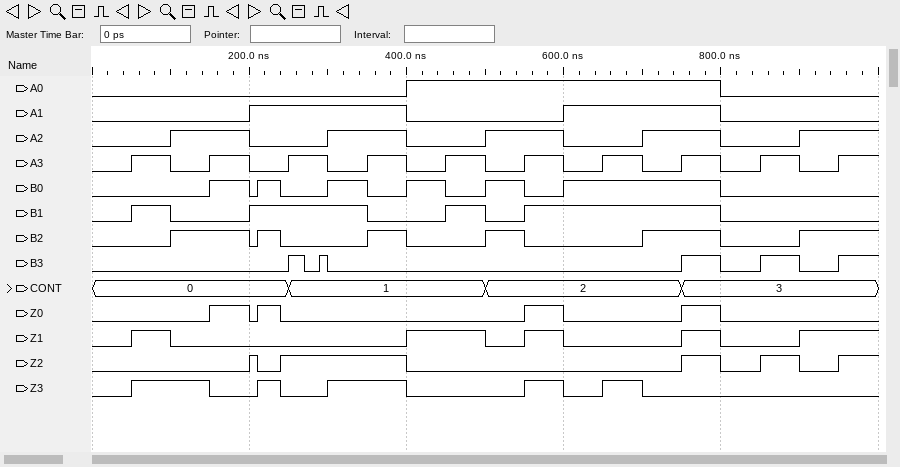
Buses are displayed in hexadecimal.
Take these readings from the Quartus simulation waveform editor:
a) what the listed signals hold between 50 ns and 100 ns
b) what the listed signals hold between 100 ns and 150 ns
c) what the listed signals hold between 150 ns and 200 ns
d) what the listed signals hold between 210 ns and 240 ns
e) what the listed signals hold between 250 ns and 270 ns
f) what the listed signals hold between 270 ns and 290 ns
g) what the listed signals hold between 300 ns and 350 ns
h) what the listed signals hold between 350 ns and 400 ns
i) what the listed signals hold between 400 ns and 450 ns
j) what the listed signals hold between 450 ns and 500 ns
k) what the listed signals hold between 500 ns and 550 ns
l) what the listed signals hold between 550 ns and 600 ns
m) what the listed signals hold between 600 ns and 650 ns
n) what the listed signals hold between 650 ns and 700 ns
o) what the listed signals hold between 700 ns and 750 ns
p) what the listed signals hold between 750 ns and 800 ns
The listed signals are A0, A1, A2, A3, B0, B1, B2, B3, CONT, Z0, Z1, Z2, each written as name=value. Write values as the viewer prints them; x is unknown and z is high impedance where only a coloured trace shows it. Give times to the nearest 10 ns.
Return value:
A0=0, A1=0, A2=0, A3=1, B0=0, B1=1, B2=0, B3=0, CONT=0, Z0=0, Z1=1, Z2=0
A0=0, A1=0, A2=1, A3=0, B0=0, B1=0, B2=1, B3=0, CONT=0, Z0=0, Z1=0, Z2=0
A0=0, A1=0, A2=1, A3=1, B0=1, B1=0, B2=1, B3=0, CONT=0, Z0=1, Z1=0, Z2=0
A0=0, A1=1, A2=0, A3=0, B0=1, B1=1, B2=1, B3=0, CONT=0, Z0=1, Z1=0, Z2=0
A0=0, A1=1, A2=0, A3=1, B0=0, B1=1, B2=0, B3=1, CONT=1, Z0=0, Z1=0, Z2=1
A0=0, A1=1, A2=0, A3=1, B0=0, B1=1, B2=0, B3=0, CONT=1, Z0=0, Z1=0, Z2=1
A0=0, A1=1, A2=1, A3=0, B0=1, B1=1, B2=0, B3=0, CONT=1, Z0=0, Z1=0, Z2=1
A0=0, A1=1, A2=1, A3=1, B0=0, B1=0, B2=1, B3=0, CONT=1, Z0=0, Z1=0, Z2=1
A0=1, A1=0, A2=0, A3=0, B0=1, B1=0, B2=0, B3=0, CONT=1, Z0=0, Z1=1, Z2=0
A0=1, A1=0, A2=0, A3=1, B0=0, B1=1, B2=0, B3=0, CONT=1, Z0=0, Z1=1, Z2=0
A0=1, A1=0, A2=1, A3=0, B0=1, B1=0, B2=1, B3=0, CONT=2, Z0=0, Z1=0, Z2=0
A0=1, A1=0, A2=1, A3=1, B0=0, B1=1, B2=0, B3=0, CONT=2, Z0=1, Z1=1, Z2=0
A0=1, A1=1, A2=0, A3=0, B0=1, B1=1, B2=0, B3=0, CONT=2, Z0=0, Z1=0, Z2=0
A0=1, A1=1, A2=0, A3=1, B0=1, B1=1, B2=0, B3=0, CONT=2, Z0=0, Z1=0, Z2=0
A0=1, A1=1, A2=1, A3=0, B0=1, B1=1, B2=1, B3=0, CONT=2, Z0=0, Z1=0, Z2=0
A0=1, A1=1, A2=1, A3=1, B0=1, B1=1, B2=1, B3=1, CONT=3, Z0=1, Z1=1, Z2=1
